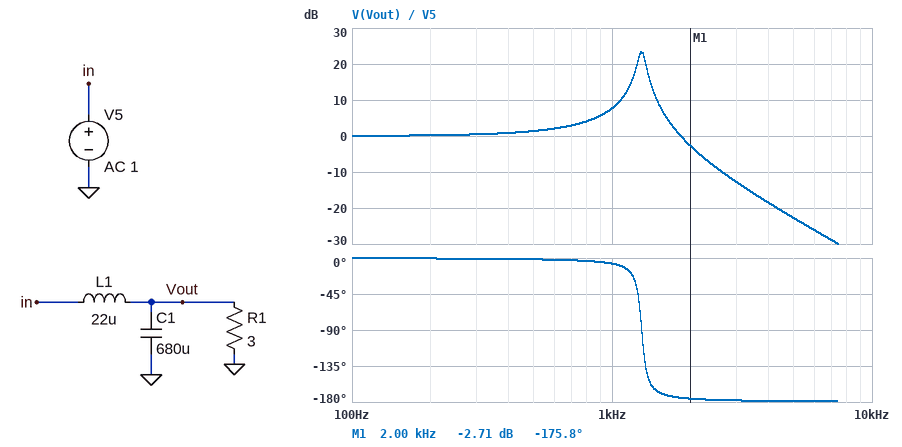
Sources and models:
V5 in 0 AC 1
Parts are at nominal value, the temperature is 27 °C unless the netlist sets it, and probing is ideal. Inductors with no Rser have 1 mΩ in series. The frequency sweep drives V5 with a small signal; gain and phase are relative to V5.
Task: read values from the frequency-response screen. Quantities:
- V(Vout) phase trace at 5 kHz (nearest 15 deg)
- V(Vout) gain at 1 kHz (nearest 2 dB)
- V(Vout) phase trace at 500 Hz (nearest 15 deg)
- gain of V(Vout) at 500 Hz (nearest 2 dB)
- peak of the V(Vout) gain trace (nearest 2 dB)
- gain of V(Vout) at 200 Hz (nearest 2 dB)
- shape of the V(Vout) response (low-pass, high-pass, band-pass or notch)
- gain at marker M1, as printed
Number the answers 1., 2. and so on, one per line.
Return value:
1. -180 deg
2. 8 dB
3. 0 deg
4. 2 dB
5. 24 dB
6. 0 dB
7. low-pass
8. -2.71 dB
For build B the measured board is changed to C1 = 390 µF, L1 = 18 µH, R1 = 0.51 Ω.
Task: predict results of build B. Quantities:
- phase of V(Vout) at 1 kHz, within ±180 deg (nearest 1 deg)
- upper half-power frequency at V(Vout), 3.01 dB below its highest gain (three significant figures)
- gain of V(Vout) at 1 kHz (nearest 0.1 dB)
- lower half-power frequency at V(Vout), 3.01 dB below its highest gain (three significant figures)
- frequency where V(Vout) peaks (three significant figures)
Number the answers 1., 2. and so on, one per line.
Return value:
1. -17 deg
2. 2.19 kHz
3. 2.4 dB
4. 1.34 kHz
5. 1.81 kHz
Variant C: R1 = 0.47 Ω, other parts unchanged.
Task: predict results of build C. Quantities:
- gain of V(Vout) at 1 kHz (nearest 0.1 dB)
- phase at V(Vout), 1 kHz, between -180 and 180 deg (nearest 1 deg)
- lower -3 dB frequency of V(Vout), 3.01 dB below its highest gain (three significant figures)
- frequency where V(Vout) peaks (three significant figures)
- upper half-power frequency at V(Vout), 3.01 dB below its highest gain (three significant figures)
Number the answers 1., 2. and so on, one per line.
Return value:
1. 5.9 dB
2. -36 deg
3. 961 Hz
4. 1.25 kHz
5. 1.49 kHz
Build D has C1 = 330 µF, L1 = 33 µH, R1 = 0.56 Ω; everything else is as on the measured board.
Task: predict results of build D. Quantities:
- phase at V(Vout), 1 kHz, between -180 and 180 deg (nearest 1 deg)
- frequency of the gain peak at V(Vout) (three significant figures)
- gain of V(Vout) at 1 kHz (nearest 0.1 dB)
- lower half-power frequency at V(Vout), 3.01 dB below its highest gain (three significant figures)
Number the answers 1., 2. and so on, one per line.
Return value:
1. -33 deg
2. 1.40 kHz
3. 3.3 dB
4. 829 Hz
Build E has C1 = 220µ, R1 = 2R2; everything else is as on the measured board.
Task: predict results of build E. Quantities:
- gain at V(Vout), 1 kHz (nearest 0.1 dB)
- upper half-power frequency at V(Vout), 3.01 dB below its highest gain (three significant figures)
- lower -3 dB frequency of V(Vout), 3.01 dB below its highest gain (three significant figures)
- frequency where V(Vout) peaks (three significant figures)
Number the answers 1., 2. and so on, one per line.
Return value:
1. 1.8 dB
2. 2.44 kHz
3. 2.10 kHz
4. 2.28 kHz
